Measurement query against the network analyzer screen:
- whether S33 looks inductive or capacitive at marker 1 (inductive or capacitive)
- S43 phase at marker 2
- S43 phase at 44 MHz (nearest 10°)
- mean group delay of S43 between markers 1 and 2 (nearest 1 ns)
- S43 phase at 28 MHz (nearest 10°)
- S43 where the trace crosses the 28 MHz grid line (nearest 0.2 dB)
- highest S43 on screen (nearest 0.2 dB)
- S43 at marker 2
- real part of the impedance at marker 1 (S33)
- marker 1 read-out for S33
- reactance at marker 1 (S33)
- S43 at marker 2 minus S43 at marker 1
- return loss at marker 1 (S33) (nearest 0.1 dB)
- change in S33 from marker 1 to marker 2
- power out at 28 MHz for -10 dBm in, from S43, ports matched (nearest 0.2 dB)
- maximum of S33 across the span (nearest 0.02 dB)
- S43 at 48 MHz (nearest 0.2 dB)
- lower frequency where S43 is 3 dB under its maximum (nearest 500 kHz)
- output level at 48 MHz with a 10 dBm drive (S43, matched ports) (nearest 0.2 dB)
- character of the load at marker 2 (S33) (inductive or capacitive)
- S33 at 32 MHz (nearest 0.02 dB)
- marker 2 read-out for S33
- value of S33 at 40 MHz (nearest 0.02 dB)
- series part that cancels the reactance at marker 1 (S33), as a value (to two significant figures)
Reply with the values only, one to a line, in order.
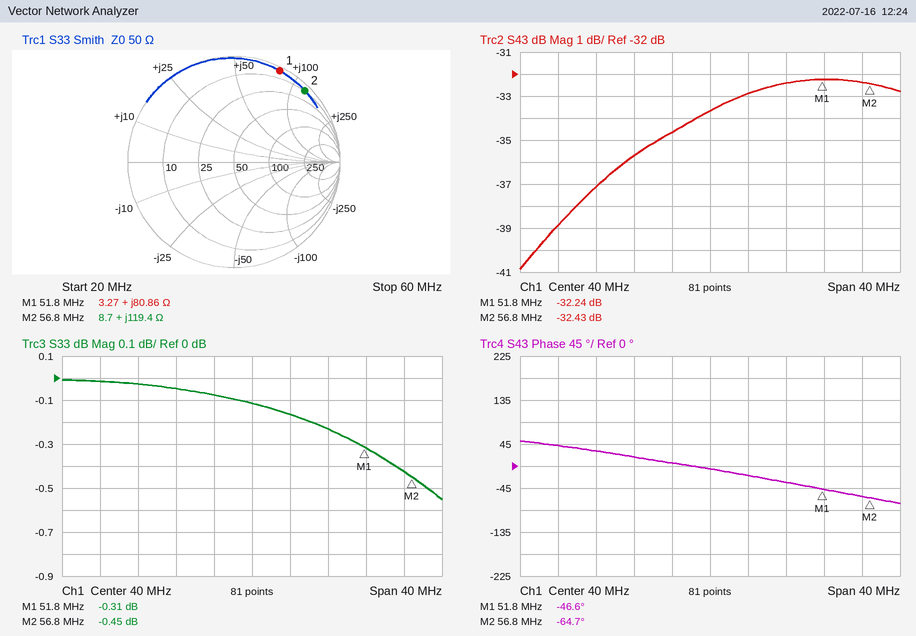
inductive
-64.7°
-20°
10 ns
30°
-37.2 dB
-32.2 dB
-32.43 dB
3.27 Ω
-0.31 dB
+80.86 Ω
-0.19 dB
0.3 dB
-0.14 dB
-47.2 dBm
0.00 dB
-32.4 dB
33.5 MHz
-22.4 dBm
inductive
-0.04 dB
-0.45 dB
-0.12 dB
38 pF
